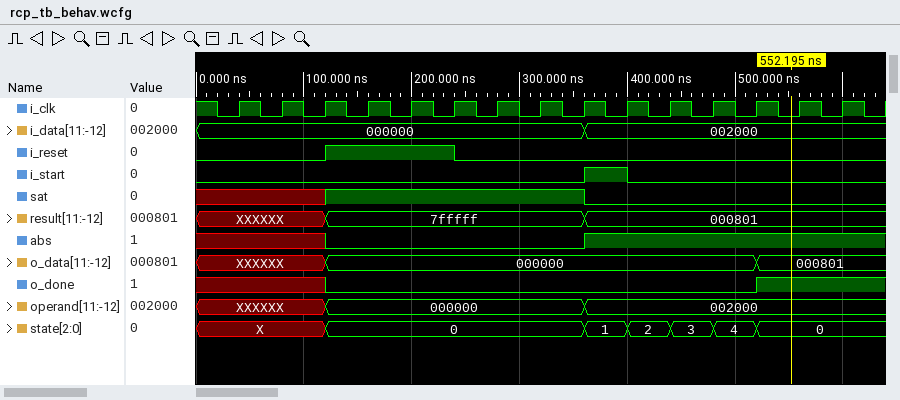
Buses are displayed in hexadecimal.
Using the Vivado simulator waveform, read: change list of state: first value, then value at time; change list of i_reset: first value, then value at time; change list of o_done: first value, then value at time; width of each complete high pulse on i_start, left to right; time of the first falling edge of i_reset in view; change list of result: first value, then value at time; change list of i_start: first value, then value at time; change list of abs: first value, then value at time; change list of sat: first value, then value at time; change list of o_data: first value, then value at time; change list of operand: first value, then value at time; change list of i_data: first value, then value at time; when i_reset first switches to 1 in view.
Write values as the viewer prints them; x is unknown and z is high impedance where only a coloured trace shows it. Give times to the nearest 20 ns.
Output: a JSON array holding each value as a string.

["X, 0 at 120 ns, 1 at 360 ns, 2 at 400 ns, 3 at 440 ns, 4 at 480 ns, 0 at 520 ns", "0, 1 at 120 ns, 0 at 240 ns", "x, 0 at 120 ns, 1 at 520 ns", "40 ns", "240 ns", "XXXXXX, 7fffff at 120 ns, 000801 at 360 ns", "0, 1 at 360 ns, 0 at 400 ns", "x, 0 at 120 ns, 1 at 360 ns", "x, 1 at 120 ns, 0 at 360 ns", "XXXXXX, 000000 at 120 ns, 000801 at 520 ns", "XXXXXX, 000000 at 120 ns, 002000 at 360 ns", "000000, 002000 at 360 ns", "120 ns"]
